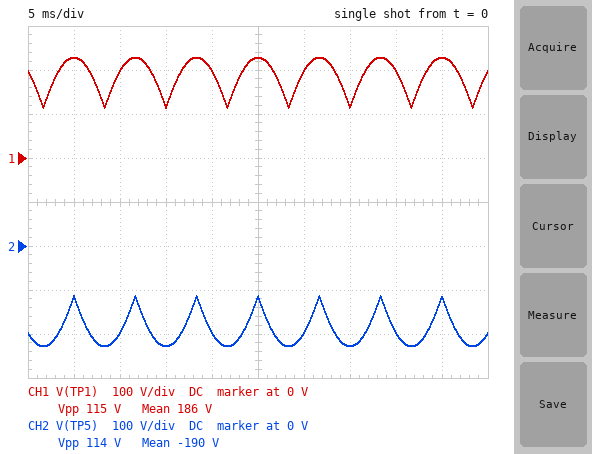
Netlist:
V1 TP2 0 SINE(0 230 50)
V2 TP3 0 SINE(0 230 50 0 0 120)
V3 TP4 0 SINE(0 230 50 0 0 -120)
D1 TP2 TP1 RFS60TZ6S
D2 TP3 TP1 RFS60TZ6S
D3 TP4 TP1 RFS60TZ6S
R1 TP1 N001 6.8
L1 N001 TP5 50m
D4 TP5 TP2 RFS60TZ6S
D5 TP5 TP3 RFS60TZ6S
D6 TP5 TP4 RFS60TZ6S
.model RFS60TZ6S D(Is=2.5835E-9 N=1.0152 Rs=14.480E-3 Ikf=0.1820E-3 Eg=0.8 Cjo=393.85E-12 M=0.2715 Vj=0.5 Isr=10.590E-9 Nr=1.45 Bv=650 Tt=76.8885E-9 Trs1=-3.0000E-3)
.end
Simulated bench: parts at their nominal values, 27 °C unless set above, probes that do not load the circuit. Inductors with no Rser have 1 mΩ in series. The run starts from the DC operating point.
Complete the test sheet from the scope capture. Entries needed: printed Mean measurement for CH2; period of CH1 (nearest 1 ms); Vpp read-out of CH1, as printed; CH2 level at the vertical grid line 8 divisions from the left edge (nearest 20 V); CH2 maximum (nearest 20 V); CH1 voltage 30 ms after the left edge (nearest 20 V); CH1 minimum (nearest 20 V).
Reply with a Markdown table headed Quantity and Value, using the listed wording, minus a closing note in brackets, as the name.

| Quantity | Value |
|---|---|
| printed Mean measurement for CH2 | -190 V |
| period of CH1 | 7 ms |
| Vpp read-out of CH1, as printed | 115 V |
| CH2 level at the vertical grid line 8 divisions from the left edge | -200 V |
| CH2 maximum | -120 V |
| CH1 voltage 30 ms after the left edge | 200 V |
| CH1 minimum | 120 V |
